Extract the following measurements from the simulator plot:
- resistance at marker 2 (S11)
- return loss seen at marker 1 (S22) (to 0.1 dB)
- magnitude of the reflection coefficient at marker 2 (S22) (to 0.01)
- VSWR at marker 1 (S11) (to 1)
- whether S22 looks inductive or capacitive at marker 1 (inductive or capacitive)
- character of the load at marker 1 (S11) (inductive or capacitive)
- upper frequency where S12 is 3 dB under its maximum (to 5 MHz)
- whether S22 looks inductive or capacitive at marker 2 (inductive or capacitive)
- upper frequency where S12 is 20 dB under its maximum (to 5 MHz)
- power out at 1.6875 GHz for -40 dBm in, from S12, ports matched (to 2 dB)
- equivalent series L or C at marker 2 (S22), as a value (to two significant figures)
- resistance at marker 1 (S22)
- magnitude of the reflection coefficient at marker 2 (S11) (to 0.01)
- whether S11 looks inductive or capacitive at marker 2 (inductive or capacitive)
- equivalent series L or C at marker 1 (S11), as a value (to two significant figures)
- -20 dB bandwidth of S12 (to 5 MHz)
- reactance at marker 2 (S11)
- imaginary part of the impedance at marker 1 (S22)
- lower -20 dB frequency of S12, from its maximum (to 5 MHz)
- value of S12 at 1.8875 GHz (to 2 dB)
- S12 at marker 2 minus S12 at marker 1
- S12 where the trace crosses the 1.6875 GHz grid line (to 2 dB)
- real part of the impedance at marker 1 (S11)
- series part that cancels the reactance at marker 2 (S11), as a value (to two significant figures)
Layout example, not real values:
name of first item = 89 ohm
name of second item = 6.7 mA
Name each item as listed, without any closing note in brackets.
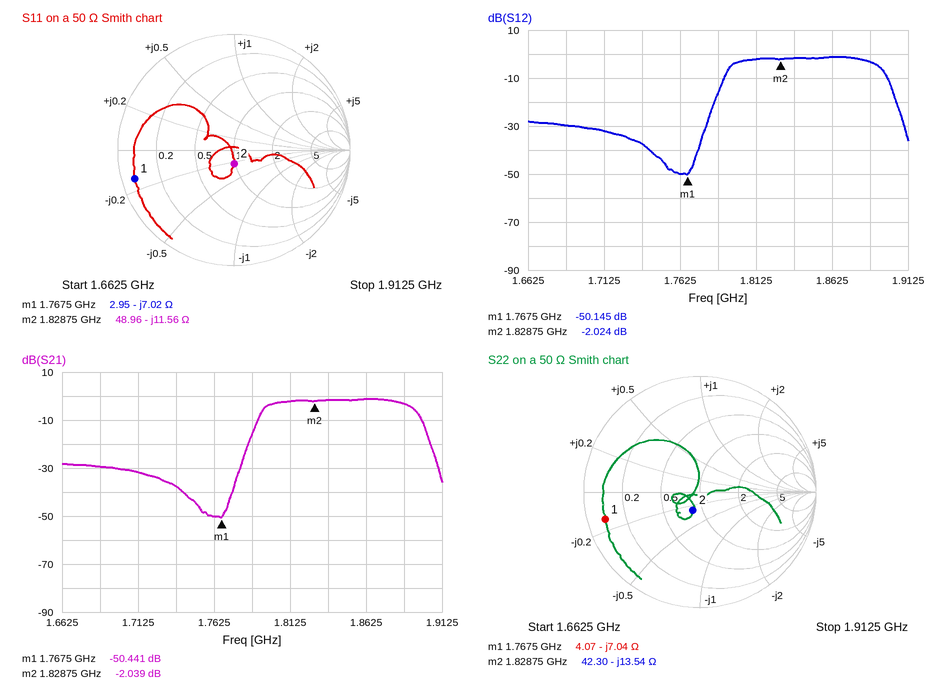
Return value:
resistance at marker 2 = 48.96 Ω
return loss seen at marker 1 (S22) = 1.4 dB
magnitude of the reflection coefficient at marker 2 (S22) = 0.17
VSWR at marker 1 (S11) = 17
whether S22 looks inductive or capacitive at marker 1 = capacitive
character of the load at marker 1 (S11) = capacitive
upper frequency where S12 is 3 dB under its maximum = 1.890 GHz
whether S22 looks inductive or capacitive at marker 2 = capacitive
upper frequency where S12 is 20 dB under its maximum = 1.905 GHz
power out at 1.6875 GHz for -40 dBm in, from S12, ports matched = -70 dBm
equivalent series L or C at marker 2 (S22), as a value = 6.4 pF
resistance at marker 1 = 4.07 Ω
magnitude of the reflection coefficient at marker 2 (S11) = 0.12
whether S11 looks inductive or capacitive at marker 2 = capacitive
equivalent series L or C at marker 1 (S11), as a value = 13 pF
-20 dB bandwidth of S12 = 120 MHz
reactance at marker 2 = -11.56 Ω
imaginary part of the impedance at marker 1 = -7.04 Ω
lower -20 dB frequency of S12, from its maximum = 1.785 GHz
value of S12 at 1.8875 GHz = -4 dB
S12 at marker 2 minus S12 at marker 1 = 48.121 dB
S12 where the trace crosses the 1.6875 GHz grid line = -30 dB
real part of the impedance at marker 1 = 2.95 Ω
series part that cancels the reactance at marker 2 (S11), as a value = 1.0 nH
